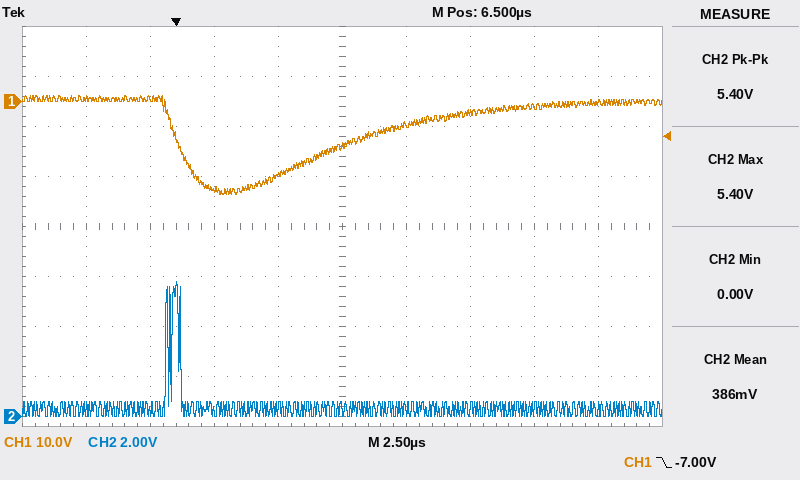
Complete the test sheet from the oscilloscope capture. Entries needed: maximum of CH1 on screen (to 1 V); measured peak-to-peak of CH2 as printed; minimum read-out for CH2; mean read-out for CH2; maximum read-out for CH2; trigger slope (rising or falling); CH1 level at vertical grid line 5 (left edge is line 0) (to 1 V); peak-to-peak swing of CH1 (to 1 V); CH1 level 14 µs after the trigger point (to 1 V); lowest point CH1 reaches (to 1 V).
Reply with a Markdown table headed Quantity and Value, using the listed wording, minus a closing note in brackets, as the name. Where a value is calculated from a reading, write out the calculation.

| Quantity | Value |
|---|---|
| maximum of CH1 on screen | 1 V |
| measured peak-to-peak of CH2 as printed | 5.40 V |
| minimum read-out for CH2 | 0.00 V |
| mean read-out for CH2 | 386 mV |
| maximum read-out for CH2 | 5.40 V |
| trigger slope | falling |
| CH1 level at vertical grid line 5 (left edge is line 0) | -9 V |
| peak-to-peak swing of CH1 | 1 V − (-19 V) = 20 V |
| CH1 level 14 µs after the trigger point | -1 V |
| lowest point CH1 reaches | -19 V |
